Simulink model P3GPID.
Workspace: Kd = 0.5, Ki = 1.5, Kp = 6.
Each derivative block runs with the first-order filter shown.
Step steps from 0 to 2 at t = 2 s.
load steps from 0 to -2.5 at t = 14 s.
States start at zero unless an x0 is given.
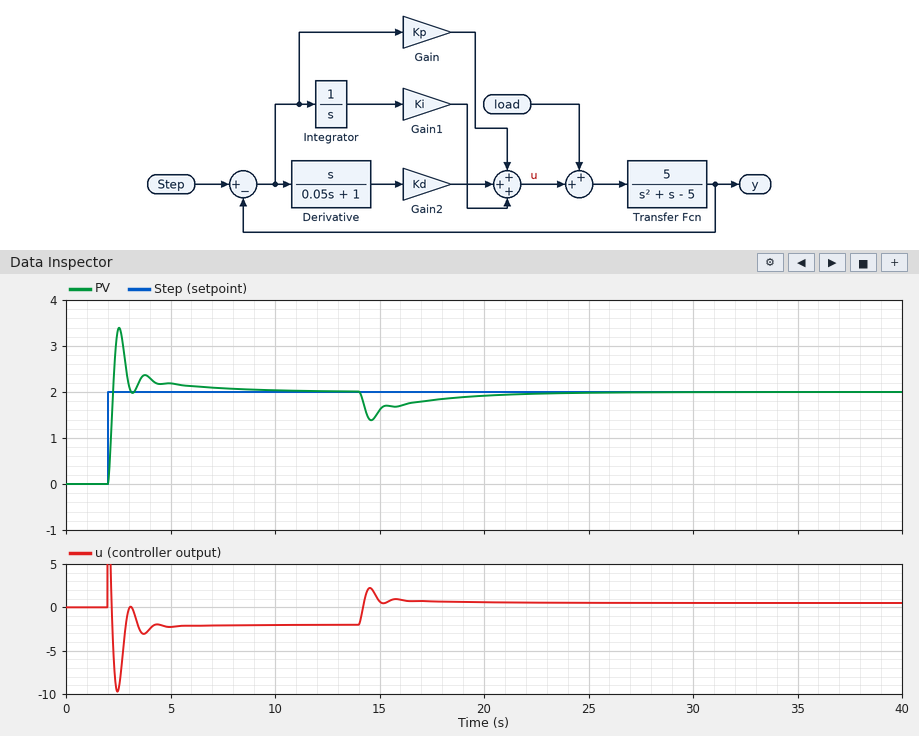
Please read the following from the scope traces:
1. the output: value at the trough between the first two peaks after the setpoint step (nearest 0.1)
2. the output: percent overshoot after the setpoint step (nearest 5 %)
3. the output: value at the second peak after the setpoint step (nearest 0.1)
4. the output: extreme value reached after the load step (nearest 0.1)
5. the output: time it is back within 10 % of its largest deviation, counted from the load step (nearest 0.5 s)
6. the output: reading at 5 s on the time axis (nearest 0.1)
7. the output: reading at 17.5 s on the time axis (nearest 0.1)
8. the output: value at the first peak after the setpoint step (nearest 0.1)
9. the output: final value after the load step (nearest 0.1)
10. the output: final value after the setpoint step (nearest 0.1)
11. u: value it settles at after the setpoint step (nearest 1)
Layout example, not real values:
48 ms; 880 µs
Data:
2.0; 70 %; 2.4; 1.4; 7.0 s; 2.2; 1.8; 3.4; 2.0; 2.0; -2
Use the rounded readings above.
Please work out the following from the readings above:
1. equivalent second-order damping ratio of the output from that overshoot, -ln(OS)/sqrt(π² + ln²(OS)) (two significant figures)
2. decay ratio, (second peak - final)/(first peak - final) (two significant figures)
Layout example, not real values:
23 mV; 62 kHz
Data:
0.11; 0.29
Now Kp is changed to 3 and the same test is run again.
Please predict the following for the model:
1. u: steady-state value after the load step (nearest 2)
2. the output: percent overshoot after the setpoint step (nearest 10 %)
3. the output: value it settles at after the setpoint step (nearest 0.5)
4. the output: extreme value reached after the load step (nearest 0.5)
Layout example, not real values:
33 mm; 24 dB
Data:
0; 80 %; 2.0; 1.0
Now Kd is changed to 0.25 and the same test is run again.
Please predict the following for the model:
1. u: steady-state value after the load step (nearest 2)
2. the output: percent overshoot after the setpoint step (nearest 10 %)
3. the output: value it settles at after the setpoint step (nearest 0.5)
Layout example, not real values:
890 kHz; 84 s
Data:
0; 90 %; 2.0
